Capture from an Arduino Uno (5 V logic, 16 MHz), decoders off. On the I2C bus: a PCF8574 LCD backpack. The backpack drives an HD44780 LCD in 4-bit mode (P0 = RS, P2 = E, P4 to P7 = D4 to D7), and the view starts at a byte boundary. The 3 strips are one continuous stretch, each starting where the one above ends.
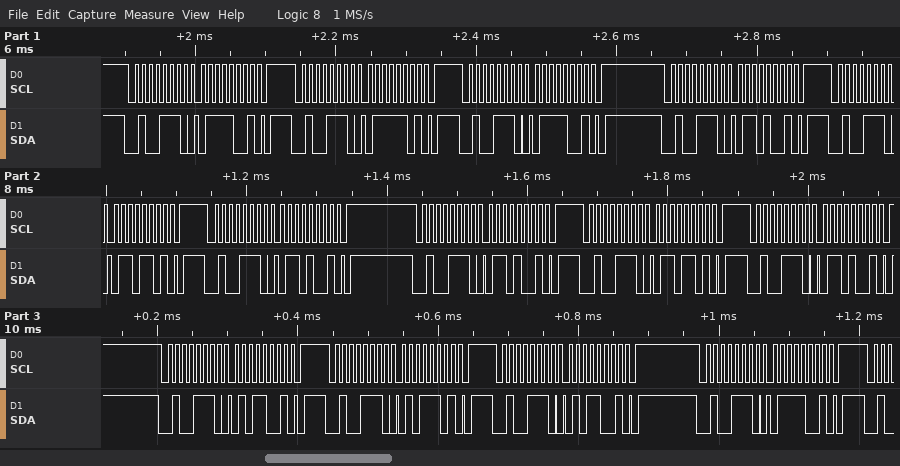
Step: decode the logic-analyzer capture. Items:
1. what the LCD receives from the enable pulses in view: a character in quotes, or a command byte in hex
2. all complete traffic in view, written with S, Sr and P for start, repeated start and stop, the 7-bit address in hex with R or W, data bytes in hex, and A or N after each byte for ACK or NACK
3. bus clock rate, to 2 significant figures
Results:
'v' 'e'
S 27W A 79 A P S 27W A 7D A P S 27W A 79 A P S 27W A 69 A P S 27W A 6D A P S 27W A 69 A P S 27W A 69 A P S 27W A 6D A P S 27W A 69 A P S 27W A 59 A P S 27W A 5D A P S 27W A 59 A P S 27W A 79 A P
100 kHz
